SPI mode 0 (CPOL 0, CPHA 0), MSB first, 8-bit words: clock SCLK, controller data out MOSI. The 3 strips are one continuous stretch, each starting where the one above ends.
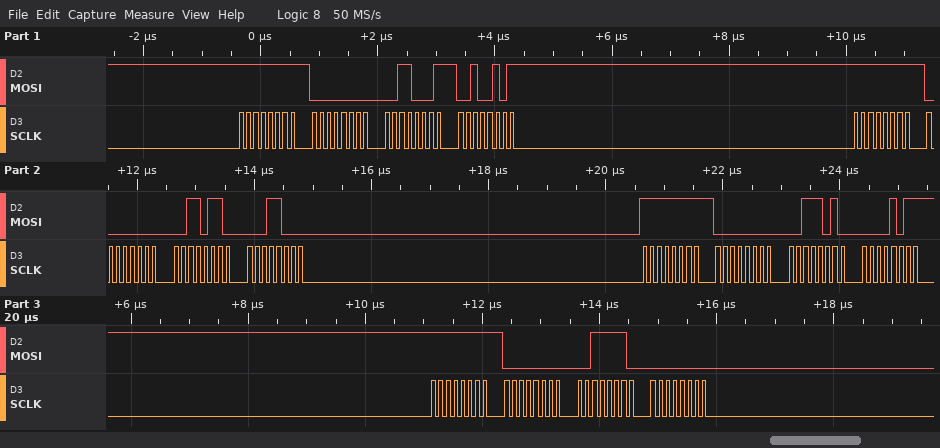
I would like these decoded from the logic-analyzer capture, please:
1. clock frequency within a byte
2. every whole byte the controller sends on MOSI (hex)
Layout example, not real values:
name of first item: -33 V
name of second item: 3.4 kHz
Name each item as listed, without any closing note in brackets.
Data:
clock frequency within a byte: 8 MHz
every whole byte the controller sends on MOSI: FF 00 31 25 FF 00 36 18 FF 00 3A 0B FF 00 3E 00
